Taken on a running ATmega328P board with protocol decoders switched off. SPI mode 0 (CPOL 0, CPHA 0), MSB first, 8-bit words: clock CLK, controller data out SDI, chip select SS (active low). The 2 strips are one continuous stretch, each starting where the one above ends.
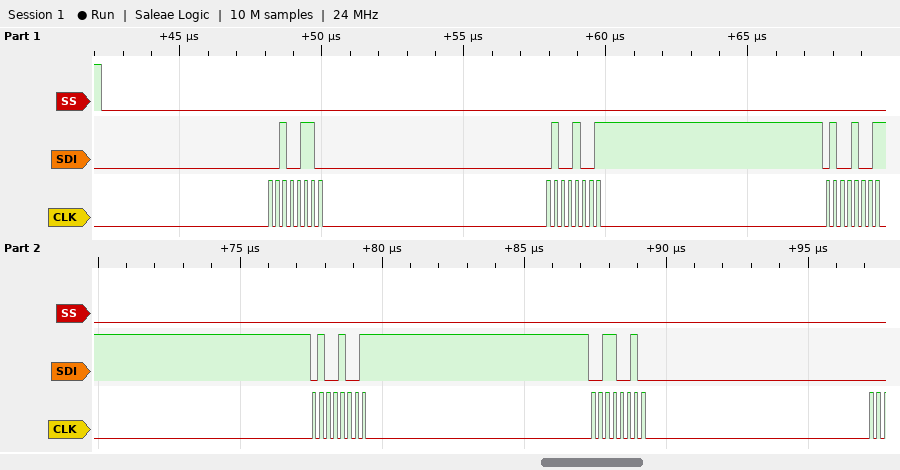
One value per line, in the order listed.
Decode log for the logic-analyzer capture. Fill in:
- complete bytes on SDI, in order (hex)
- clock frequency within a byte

26 49 49 49 32
4 MHz
